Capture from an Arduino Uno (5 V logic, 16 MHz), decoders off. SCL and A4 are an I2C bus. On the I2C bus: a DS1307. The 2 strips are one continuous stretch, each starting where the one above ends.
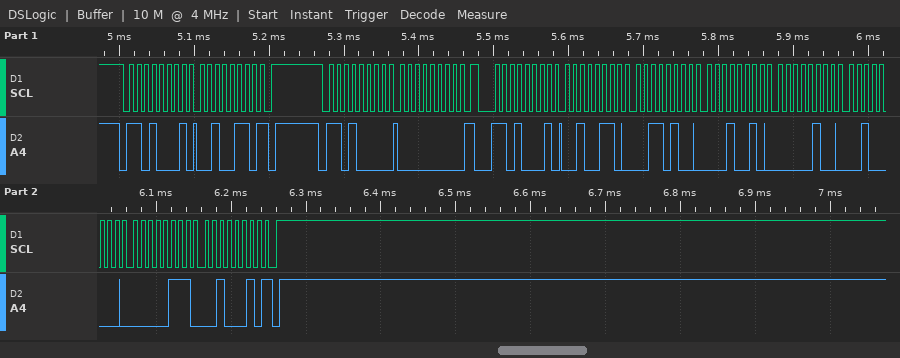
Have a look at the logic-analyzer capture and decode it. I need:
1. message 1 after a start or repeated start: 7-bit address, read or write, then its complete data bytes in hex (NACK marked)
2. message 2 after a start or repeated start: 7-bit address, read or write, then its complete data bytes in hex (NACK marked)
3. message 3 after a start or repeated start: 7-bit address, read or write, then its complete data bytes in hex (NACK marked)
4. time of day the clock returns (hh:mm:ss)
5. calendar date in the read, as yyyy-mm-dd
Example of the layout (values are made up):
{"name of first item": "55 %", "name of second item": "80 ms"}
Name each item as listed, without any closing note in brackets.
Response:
{"message 1 after a start or repeated start: 7-bit address, read or write, then its complete data bytes in hex": "0x68 read: 26 NACK", "message 2 after a start or repeated start: 7-bit address, read or write, then its complete data bytes in hex": "0x68 write: 00", "message 3 after a start or repeated start: 7-bit address, read or write, then its complete data bytes in hex": "0x68 read: 26 34 12 04 20 07 22 NACK", "time of day the clock returns": "12:34:26", "calendar date in the read, as yyyy-mm-dd": "2022-07-20"}
